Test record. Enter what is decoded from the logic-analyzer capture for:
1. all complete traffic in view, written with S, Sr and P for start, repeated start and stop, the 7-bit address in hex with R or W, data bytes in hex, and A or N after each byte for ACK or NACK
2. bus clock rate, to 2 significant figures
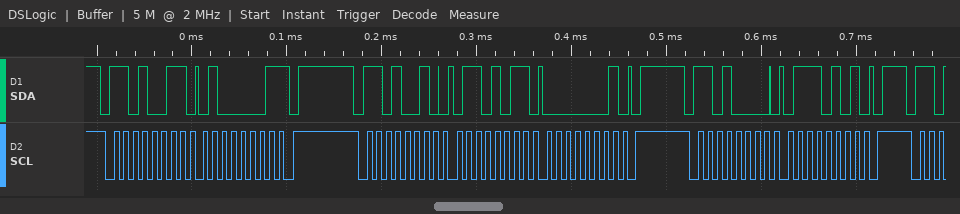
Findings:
S 69R A 41 N P S 69W A 6B A 01 A P S 68W A 75 A P
100 kHz
